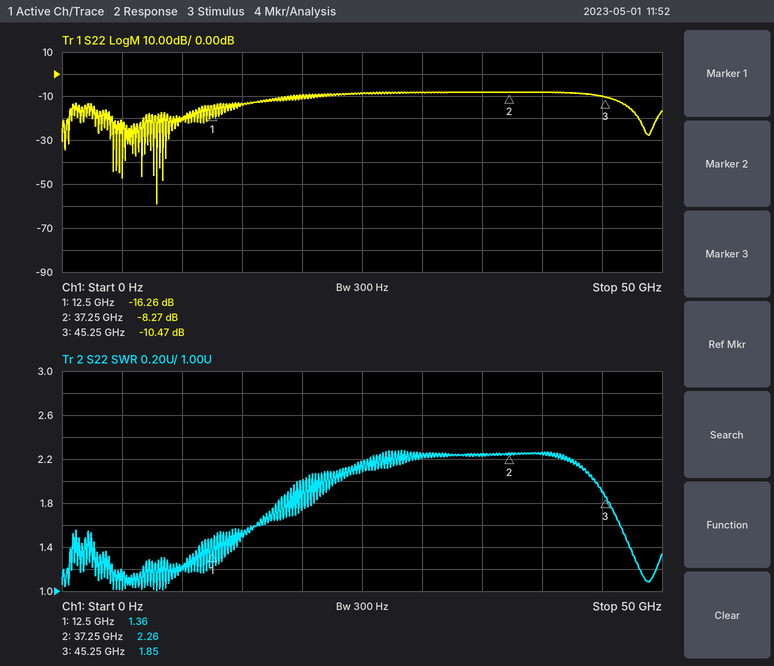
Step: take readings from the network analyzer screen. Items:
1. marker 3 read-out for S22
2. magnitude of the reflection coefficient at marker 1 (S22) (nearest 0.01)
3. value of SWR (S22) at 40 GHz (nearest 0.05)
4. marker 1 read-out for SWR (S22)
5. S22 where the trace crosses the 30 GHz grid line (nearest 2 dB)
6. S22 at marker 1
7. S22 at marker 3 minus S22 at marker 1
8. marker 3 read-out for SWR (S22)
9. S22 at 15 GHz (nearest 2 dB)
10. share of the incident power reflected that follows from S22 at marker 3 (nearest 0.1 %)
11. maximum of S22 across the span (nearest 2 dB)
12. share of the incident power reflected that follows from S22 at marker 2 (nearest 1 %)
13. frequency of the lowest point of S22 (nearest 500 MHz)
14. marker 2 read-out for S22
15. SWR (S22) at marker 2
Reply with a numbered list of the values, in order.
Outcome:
1. -10.47 dB
2. 0.15
3. 2.25
4. 1.36
5. -8 dB
6. -16.26 dB
7. 5.79 dB
8. 1.85
9. -14 dB
10. 9.0 %
11. -8 dB
12. 15 %
13. 8.0 GHz
14. -8.27 dB
15. 2.26
